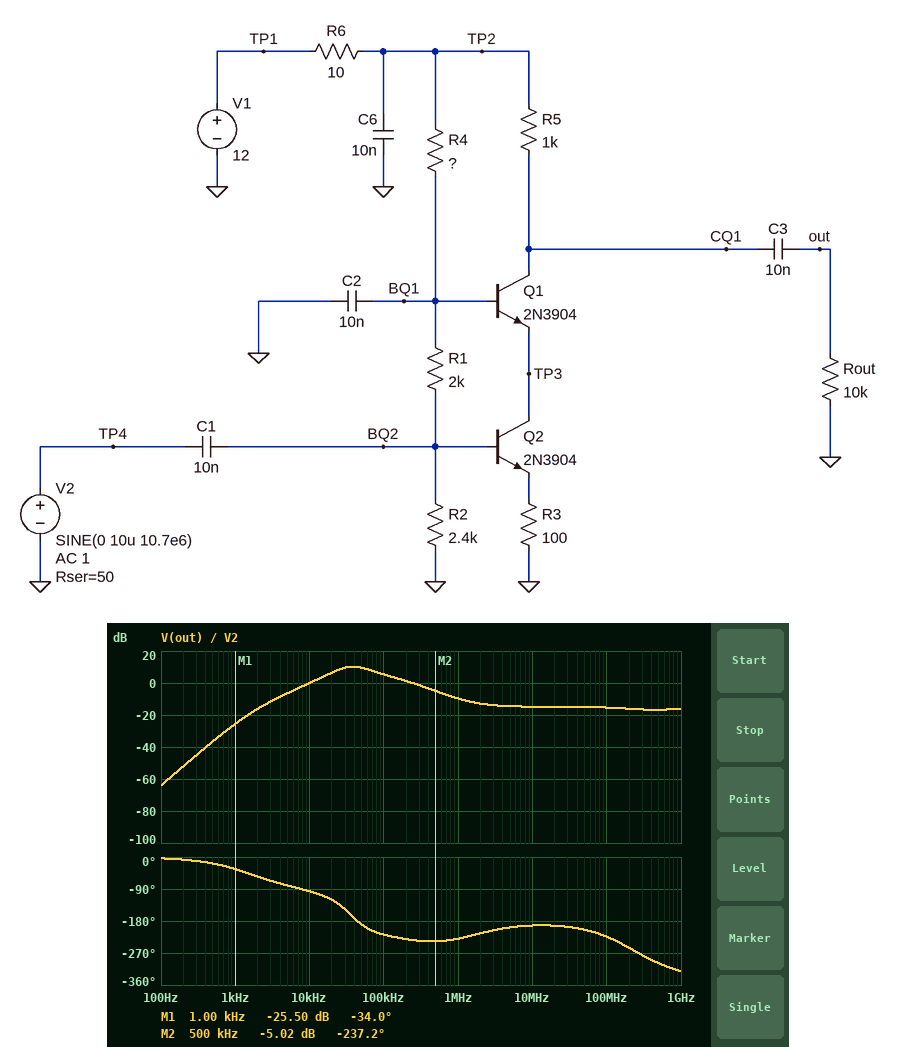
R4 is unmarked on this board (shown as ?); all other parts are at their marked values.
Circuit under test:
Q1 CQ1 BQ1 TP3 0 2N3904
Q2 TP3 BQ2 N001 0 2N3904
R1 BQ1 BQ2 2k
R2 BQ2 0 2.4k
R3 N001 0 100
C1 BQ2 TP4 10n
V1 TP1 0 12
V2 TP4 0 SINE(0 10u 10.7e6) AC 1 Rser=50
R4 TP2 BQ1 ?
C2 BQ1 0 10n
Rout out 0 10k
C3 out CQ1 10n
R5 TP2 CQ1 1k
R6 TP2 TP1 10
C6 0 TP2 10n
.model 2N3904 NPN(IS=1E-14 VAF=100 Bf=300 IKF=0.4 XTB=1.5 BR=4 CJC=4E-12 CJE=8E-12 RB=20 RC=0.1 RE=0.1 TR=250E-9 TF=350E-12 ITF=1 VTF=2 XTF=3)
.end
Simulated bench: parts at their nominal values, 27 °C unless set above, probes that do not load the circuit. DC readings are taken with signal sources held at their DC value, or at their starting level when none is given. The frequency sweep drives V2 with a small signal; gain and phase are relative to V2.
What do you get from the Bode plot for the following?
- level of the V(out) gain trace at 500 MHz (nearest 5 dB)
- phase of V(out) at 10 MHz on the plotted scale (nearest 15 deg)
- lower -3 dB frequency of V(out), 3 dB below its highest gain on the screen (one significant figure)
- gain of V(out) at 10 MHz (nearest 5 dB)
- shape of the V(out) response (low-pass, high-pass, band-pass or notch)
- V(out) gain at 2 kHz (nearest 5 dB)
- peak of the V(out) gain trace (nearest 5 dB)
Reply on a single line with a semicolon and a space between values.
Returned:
-15 dB; -195 deg; 20 kHz; -15 dB; band-pass; -15 dB; 10 dB
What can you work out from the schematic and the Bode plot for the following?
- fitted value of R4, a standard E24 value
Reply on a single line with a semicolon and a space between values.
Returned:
8.2 kΩ
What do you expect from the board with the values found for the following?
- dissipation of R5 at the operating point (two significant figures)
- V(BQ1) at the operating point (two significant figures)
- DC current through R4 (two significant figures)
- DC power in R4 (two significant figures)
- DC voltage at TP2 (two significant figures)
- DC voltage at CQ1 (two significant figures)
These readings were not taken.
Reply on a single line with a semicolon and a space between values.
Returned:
88 mW; 3.2 V; 1.1 mA; 9.3 mW; 12 V; 2.5 V
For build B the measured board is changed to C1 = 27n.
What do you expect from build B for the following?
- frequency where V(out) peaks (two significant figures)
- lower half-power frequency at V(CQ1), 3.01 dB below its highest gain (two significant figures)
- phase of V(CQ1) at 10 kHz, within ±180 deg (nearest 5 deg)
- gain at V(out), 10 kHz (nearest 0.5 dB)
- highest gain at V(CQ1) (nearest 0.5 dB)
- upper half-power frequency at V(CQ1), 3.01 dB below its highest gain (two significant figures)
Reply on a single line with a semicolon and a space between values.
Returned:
23 kHz; 11 kHz; -125 deg; 8.0 dB; 12.0 dB; 50 kHz
